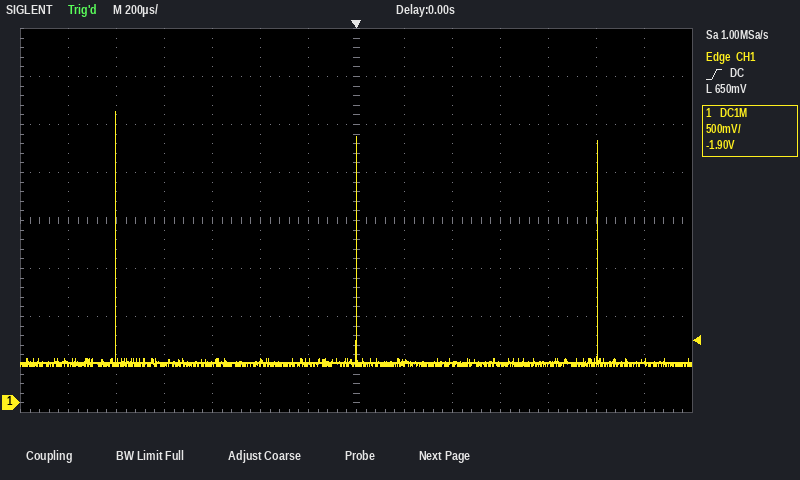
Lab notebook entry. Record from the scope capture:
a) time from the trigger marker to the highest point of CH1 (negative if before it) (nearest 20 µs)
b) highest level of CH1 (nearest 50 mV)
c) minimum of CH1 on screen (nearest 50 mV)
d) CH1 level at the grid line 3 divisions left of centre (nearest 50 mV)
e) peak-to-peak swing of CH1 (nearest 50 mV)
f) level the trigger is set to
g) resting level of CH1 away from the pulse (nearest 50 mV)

-1.00 ms
3.05 V
400 mV
400 mV
2.65 V
650 mV
400 mV
